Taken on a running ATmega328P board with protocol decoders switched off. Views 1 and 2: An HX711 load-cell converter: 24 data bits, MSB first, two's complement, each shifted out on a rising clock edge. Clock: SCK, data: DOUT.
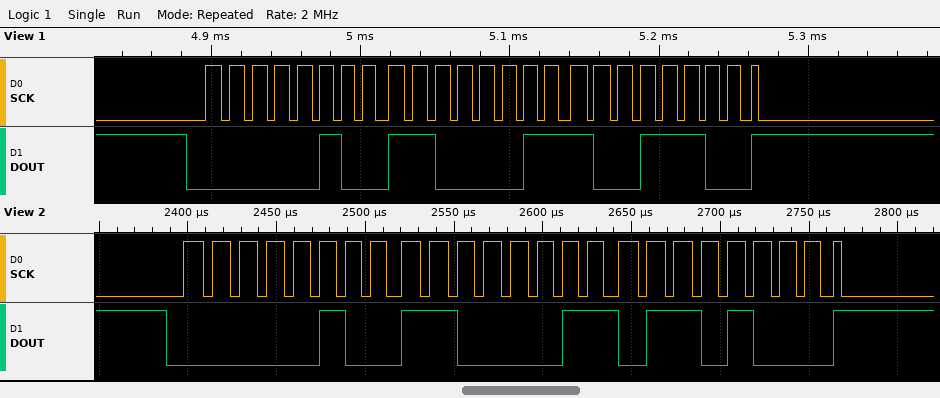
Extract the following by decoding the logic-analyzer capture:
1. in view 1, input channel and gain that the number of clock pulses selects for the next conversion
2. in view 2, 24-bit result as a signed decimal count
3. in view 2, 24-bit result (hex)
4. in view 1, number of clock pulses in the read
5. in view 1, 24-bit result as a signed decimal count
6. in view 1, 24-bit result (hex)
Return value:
channel A, gain 128
312168
0x04C368
25
312220
0x04C39C
